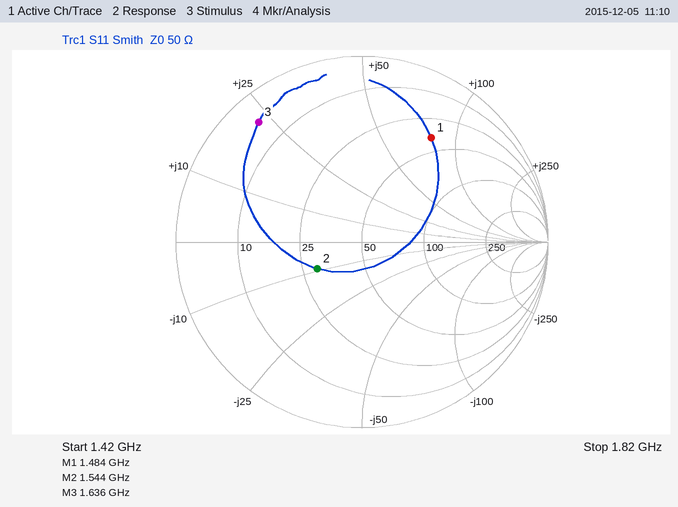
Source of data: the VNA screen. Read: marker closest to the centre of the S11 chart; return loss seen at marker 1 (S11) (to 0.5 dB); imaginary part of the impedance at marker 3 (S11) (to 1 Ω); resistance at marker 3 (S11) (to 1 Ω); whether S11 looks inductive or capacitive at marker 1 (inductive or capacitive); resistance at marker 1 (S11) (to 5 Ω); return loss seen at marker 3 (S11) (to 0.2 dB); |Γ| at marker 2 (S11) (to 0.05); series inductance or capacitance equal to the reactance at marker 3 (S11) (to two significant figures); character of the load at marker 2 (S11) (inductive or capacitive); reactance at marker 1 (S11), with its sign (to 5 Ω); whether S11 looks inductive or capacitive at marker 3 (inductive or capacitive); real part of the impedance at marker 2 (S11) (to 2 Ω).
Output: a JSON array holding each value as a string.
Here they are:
["marker 2", "3.5 dB", "+23 Ω", "5 Ω", "inductive", "40 Ω", "1.4 dB", "0.30", "2.2 nH", "capacitive", "+80 Ω", "inductive", "30 Ω"]
